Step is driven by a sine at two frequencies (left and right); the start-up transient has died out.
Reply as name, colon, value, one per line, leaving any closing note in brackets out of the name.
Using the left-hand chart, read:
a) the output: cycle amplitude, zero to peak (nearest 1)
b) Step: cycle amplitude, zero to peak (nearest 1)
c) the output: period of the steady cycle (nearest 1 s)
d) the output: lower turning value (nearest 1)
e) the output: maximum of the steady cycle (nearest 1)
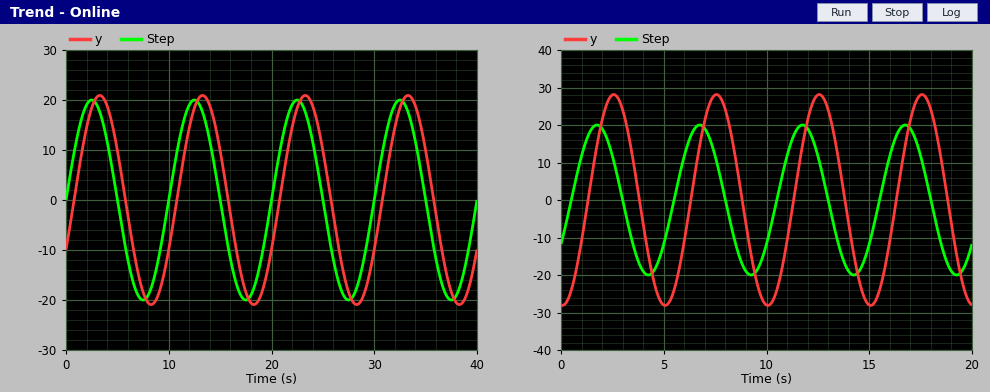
the output: cycle amplitude, zero to peak: 21
Step: cycle amplitude, zero to peak: 20
the output: period of the steady cycle: 10 s
the output: lower turning value: -21
the output: maximum of the steady cycle: 21
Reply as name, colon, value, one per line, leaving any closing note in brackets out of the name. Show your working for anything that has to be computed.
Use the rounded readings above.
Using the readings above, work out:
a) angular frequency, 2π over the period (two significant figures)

angular frequency, 2π over the period: 2π / 10 = 0.63 rad/s
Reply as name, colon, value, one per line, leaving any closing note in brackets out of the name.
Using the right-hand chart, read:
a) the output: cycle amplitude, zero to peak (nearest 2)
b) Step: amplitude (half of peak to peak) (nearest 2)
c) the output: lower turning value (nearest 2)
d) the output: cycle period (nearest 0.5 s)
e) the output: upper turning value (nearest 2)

the output: cycle amplitude, zero to peak: 28
Step: amplitude (half of peak to peak): 20
the output: lower turning value: -28
the output: cycle period: 5.0 s
the output: upper turning value: 28
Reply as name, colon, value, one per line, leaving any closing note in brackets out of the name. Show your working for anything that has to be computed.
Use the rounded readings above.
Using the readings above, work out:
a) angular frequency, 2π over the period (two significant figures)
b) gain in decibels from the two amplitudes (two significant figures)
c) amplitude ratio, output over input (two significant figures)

angular frequency, 2π over the period: 2π / 5 = 1.3 rad/s
gain in decibels from the two amplitudes: 20 log10(28 / 20) = 2.9 dB
amplitude ratio, output over input: 28 / 20 = 1.4
